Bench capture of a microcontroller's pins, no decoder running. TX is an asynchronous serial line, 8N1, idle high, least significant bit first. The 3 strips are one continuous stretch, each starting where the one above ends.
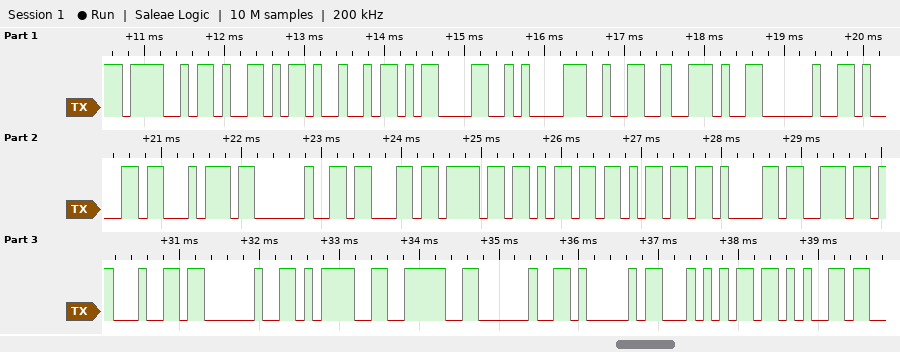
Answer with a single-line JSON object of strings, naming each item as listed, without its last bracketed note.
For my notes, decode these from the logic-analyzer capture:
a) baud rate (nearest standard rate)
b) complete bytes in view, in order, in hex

{"baud rate": "9600 baud", "complete bytes in view, in order, in hex": "4F 59 49 0D 0A 32 2E 20 61 74 20 63 6F 6D 6D 61 6E 64 20 3D 3E 20 41 54 2B"}
